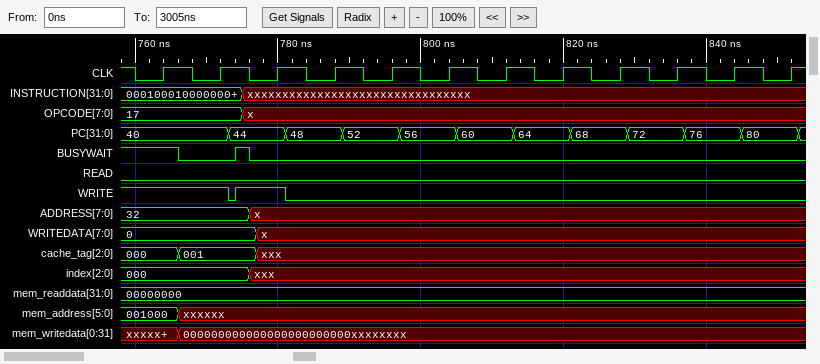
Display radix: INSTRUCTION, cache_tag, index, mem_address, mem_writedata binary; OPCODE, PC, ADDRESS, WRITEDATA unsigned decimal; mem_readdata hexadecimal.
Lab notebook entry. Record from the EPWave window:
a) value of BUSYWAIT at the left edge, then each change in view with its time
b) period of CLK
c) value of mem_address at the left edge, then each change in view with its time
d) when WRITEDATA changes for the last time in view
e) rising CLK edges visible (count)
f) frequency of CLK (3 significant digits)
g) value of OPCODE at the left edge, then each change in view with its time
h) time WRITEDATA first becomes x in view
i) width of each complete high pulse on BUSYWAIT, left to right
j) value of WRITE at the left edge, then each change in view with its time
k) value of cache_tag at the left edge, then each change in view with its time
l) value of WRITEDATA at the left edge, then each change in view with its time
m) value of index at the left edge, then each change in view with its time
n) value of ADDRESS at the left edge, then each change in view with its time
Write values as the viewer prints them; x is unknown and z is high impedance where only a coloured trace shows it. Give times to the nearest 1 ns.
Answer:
1, 0 at 766 ns, 1 at 774 ns, 0 at 776 ns
8 ns
001000, xxxxxx at 766 ns
777 ns
12
125 MHz
17, x at 775 ns
777 ns
2 ns
1, 0 at 773 ns, 1 at 774 ns, 0 at 781 ns
000, 001 at 766 ns, xxx at 777 ns
0, x at 777 ns
000, xxx at 776 ns
32, x at 776 ns
